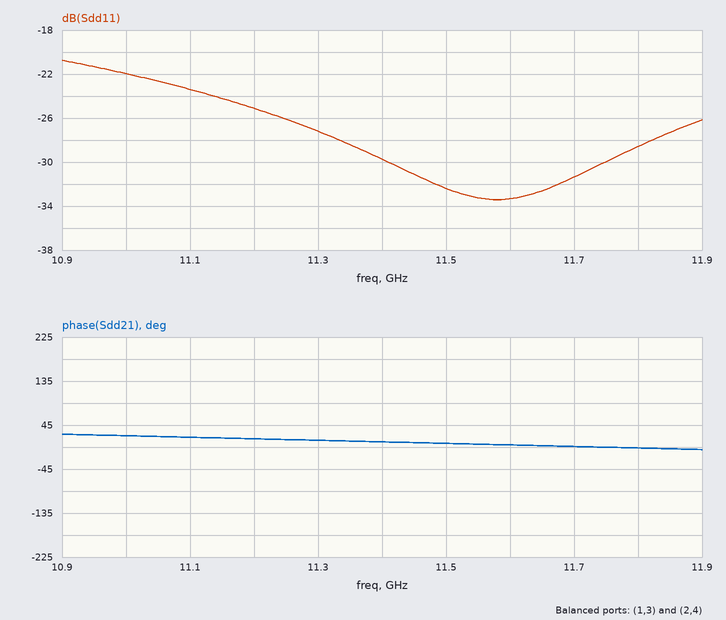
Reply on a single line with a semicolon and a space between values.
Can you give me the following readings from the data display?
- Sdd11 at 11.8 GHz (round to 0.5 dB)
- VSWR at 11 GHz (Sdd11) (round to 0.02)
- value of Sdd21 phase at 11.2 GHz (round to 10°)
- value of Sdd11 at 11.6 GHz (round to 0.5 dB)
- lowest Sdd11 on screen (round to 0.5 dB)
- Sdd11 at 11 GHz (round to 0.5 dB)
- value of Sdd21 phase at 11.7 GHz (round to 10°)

-28.5 dB; 1.18; 20°; -33.5 dB; -33.5 dB; -22.0 dB; 0°
